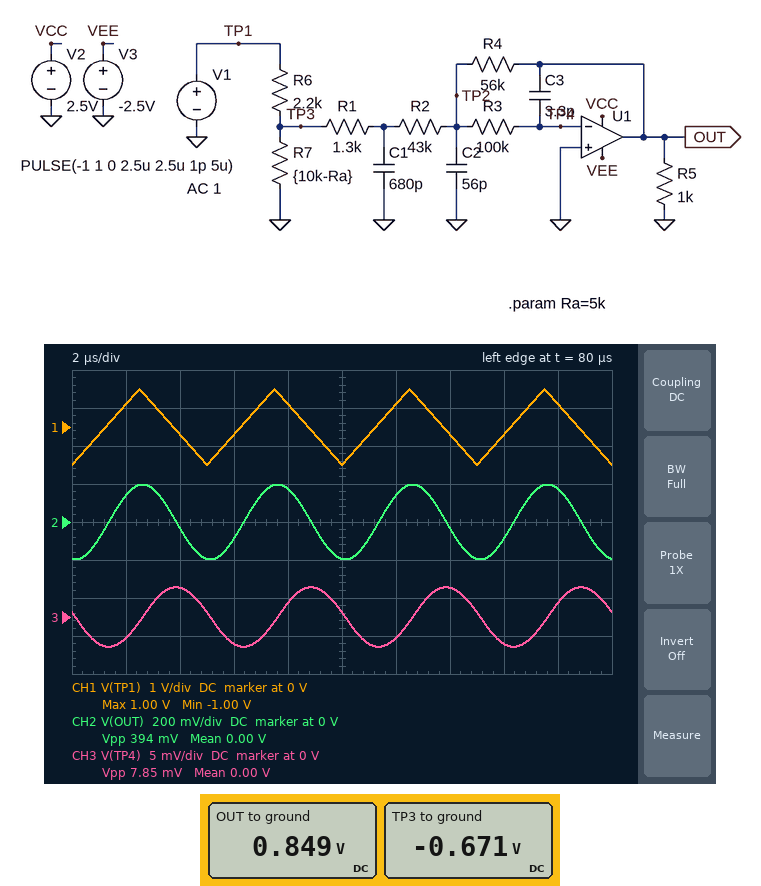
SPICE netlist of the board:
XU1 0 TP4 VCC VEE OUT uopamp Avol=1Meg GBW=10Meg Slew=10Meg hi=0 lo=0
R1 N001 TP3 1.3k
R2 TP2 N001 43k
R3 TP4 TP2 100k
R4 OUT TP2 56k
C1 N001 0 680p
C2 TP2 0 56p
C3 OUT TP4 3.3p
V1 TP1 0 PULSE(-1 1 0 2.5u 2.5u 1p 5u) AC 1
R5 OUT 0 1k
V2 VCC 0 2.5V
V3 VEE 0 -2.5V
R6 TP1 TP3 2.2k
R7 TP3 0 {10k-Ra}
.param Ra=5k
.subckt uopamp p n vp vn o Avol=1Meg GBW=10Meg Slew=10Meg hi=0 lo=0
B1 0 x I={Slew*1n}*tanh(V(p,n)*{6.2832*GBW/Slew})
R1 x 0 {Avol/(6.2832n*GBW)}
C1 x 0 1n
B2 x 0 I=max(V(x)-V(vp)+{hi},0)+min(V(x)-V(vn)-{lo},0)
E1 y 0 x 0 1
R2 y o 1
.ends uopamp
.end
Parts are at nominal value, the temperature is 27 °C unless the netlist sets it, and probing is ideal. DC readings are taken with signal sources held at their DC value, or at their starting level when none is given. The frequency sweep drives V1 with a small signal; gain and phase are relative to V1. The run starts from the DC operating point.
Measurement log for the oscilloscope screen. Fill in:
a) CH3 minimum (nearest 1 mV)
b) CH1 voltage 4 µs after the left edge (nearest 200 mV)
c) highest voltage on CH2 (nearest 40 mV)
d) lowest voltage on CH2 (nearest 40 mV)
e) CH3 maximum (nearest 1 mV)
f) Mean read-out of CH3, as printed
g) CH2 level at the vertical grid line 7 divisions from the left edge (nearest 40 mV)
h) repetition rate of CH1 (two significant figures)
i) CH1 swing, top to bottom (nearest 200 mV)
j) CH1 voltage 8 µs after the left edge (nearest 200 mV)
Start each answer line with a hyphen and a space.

- -4 mV
- -200 mV
- 200 mV
- -200 mV
- 4 mV
- 0.00 V
- -40 mV
- 200 kHz
- 2.0 V
- 600 mV
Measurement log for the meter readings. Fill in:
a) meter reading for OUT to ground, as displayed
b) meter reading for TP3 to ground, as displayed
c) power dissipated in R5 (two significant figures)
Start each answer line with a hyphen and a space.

- 0.849 V
- -0.671 V
- 720 µW
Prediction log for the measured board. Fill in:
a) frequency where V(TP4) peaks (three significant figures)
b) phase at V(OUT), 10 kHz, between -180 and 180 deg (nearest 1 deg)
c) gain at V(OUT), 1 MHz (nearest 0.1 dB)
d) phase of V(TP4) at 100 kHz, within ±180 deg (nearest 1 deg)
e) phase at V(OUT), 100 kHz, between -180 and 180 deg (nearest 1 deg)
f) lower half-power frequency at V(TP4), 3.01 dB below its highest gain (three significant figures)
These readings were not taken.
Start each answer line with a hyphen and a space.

- 129 kHz
- 170 deg
- -55.1 dB
- -6 deg
- 84 deg
- 71.1 kHz
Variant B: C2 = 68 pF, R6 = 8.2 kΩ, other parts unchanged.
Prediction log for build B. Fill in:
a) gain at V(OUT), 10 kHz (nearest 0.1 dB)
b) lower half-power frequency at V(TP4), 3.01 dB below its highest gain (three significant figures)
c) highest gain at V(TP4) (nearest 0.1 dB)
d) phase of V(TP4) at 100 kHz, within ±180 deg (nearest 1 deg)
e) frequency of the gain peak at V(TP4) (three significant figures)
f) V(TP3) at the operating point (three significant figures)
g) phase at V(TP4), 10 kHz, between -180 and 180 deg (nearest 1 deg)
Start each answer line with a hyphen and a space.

- -7.1 dB
- 62.4 kHz
- -50.2 dB
- -22 deg
- 117 kHz
- -354 mV
- 77 deg
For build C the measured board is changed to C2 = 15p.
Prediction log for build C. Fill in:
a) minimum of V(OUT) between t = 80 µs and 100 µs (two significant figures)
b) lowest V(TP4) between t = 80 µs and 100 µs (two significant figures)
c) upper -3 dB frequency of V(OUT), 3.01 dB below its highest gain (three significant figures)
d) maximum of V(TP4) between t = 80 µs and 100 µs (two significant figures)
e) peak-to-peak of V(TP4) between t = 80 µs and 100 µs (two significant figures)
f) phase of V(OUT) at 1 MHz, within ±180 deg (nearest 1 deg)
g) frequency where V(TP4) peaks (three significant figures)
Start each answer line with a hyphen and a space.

- -210 mV
- -4.4 mV
- 81.6 kHz
- 4.4 mV
- 8.7 mV
- -60 deg
- 140 kHz
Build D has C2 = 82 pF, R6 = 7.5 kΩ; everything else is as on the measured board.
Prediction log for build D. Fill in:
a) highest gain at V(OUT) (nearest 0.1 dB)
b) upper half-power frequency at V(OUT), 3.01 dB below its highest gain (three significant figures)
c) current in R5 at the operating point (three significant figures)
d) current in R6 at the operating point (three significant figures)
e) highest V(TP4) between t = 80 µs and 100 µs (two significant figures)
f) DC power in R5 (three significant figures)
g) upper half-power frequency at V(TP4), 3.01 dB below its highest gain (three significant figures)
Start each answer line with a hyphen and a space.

- -6.5 dB
- 106 kHz
- 474 µA
- 83.4 µA
- 1.1 mV
- 224 µW
- 154 kHz
